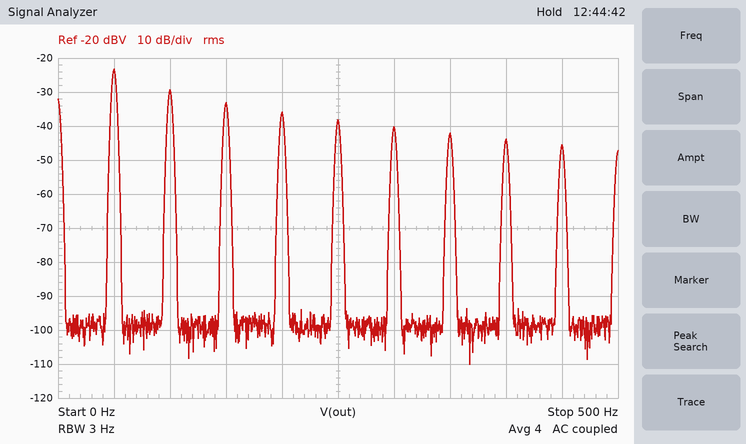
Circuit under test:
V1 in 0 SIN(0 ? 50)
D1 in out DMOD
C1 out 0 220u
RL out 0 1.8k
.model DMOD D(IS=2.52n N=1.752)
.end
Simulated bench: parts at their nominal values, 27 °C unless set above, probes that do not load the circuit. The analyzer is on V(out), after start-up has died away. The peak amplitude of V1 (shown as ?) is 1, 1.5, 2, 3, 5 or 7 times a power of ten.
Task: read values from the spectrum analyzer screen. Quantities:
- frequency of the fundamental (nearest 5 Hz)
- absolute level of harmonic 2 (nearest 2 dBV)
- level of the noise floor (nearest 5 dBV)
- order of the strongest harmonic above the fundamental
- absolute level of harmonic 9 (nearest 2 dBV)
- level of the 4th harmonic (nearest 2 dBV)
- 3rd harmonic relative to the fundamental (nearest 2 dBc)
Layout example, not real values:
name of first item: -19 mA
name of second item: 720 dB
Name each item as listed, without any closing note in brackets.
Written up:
frequency of the fundamental: 50 Hz
absolute level of harmonic 2: -30 dBV
level of the noise floor: -100 dBV
order of the strongest harmonic above the fundamental: 2
absolute level of harmonic 9: -46 dBV
level of the 4th harmonic: -36 dBV
3rd harmonic relative to the fundamental: -10 dBc
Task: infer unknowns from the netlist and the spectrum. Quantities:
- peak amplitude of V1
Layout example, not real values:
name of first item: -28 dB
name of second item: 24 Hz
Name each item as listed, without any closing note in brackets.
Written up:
peak amplitude of V1: 7 V
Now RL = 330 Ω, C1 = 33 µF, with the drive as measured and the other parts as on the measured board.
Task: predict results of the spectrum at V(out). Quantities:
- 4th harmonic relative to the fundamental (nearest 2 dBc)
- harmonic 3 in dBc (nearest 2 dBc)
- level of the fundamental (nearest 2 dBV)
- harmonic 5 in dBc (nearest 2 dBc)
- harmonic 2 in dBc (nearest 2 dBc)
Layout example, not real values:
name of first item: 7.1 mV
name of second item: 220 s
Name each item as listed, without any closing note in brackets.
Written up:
4th harmonic relative to the fundamental: -22 dBc
harmonic 3 in dBc: -14 dBc
level of the fundamental: 2 dBV
harmonic 5 in dBc: -28 dBc
harmonic 2 in dBc: -8 dBc
